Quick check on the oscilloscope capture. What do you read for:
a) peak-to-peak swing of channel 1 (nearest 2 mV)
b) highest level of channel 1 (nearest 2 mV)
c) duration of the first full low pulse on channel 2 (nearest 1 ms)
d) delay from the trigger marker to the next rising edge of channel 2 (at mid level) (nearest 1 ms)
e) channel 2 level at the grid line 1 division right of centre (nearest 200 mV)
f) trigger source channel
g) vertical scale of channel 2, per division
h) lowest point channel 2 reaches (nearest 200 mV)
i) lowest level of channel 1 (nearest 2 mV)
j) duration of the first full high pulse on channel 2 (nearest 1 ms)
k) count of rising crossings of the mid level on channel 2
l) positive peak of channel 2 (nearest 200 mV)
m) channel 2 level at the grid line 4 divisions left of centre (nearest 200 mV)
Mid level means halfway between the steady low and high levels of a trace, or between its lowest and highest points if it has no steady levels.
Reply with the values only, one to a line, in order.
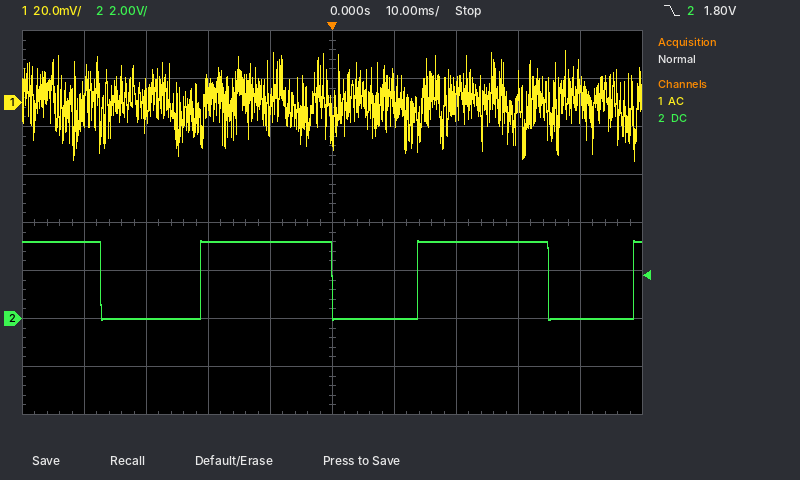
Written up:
46 mV
22 mV
16 ms
14 ms
0.0 V
channel 2
2 V
0.0 V
-24 mV
21 ms
3
3.2 V
3.2 V
